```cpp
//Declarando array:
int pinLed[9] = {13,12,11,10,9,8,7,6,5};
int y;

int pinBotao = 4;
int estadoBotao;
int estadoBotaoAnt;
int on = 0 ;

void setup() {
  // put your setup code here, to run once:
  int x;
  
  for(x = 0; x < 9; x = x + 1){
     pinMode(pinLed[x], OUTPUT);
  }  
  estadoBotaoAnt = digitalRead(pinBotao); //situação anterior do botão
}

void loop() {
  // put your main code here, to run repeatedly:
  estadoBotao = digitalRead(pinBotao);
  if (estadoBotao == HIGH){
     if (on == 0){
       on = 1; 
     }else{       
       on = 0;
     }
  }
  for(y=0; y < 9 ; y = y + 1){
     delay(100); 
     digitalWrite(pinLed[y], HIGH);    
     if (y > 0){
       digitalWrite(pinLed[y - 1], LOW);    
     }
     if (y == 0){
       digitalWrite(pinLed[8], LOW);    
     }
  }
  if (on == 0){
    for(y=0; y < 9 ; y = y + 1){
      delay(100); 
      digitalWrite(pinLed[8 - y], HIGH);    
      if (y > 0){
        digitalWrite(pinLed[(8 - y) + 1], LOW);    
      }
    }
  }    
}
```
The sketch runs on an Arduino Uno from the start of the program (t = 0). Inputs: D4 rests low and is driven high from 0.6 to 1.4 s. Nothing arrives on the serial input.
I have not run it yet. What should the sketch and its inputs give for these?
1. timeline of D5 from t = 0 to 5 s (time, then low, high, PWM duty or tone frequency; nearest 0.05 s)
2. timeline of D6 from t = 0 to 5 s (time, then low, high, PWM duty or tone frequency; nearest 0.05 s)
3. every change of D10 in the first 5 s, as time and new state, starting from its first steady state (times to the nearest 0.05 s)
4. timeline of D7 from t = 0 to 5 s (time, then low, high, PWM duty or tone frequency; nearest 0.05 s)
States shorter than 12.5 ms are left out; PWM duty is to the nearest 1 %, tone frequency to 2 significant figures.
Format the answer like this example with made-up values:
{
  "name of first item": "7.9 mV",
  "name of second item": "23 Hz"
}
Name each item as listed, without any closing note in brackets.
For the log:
{
  "timeline of D5 from t = 0 to 5 s": "0 s low; 0.9 s high; 1.1 s low; 2.7 s high; 2.9 s low; 4.5 s high; 4.7 s low",
  "timeline of D6 from t = 0 to 5 s": "0 s low; 0.8 s high; 0.9 s low; 1.1 s high; 1.2 s low; 2.6 s high; 2.7 s low; 2.9 s high; 3 s low; 4.4 s high; 4.5 s low; 4.7 s high; 4.8 s low",
  "every change of D10 in the first 5 s, as time and new state, starting from its first steady state": "0 s low; 0.4 s high; 0.5 s low; 1.5 s high; 1.6 s low; 2.2 s high; 2.3 s low; 3.3 s high; 3.4 s low; 4 s high; 4.1 s low",
  "timeline of D7 from t = 0 to 5 s": "0 s low; 0.7 s high; 0.8 s low; 1.2 s high; 1.3 s low; 2.5 s high; 2.6 s low; 3 s high; 3.1 s low; 4.3 s high; 4.4 s low; 4.8 s high; 4.9 s low"
}
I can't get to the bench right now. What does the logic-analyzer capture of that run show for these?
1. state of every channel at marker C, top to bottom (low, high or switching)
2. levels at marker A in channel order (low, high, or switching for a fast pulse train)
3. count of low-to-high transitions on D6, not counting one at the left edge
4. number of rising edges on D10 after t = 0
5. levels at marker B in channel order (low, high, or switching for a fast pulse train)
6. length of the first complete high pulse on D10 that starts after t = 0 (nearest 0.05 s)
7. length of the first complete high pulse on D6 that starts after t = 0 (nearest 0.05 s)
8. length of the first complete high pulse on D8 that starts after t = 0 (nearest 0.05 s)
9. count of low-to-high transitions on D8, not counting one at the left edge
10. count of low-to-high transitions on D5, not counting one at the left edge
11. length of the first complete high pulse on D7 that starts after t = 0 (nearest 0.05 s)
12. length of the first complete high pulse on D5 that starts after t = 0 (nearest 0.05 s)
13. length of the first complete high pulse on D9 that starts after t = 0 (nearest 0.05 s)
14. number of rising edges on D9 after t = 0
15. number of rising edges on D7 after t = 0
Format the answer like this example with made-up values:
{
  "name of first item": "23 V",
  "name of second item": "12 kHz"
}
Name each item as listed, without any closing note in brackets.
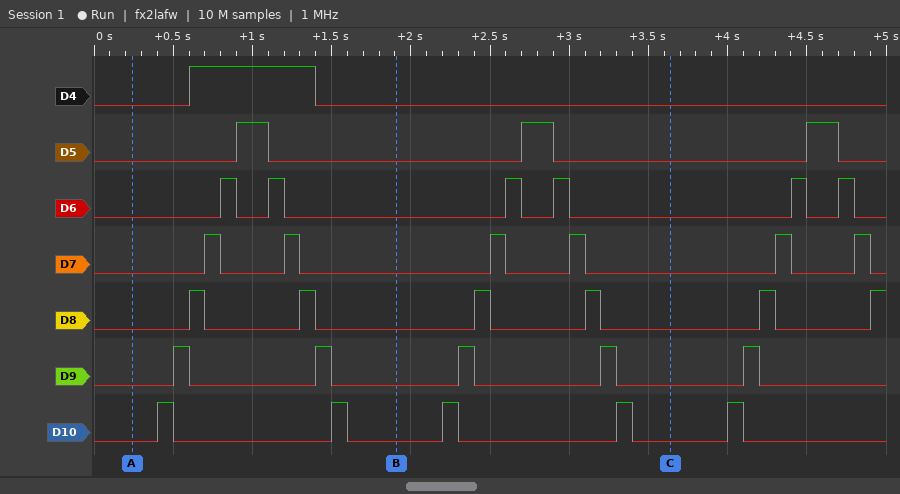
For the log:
{
  "state of every channel at marker C, top to bottom": "D4 low, D5 low, D6 low, D7 low, D8 low, D9 low, D10 low",
  "levels at marker A in channel order": "D4 low, D5 low, D6 low, D7 low, D8 low, D9 low, D10 low",
  "count of low-to-high transitions on D6, not counting one at the left edge": "6",
  "number of rising edges on D10 after t = 0": "5",
  "levels at marker B in channel order": "D4 low, D5 low, D6 low, D7 low, D8 low, D9 low, D10 low",
  "length of the first complete high pulse on D10 that starts after t = 0": "0.10 s",
  "length of the first complete high pulse on D6 that starts after t = 0": "0.10 s",
  "length of the first complete high pulse on D8 that starts after t = 0": "0.10 s",
  "count of low-to-high transitions on D8, not counting one at the left edge": "6",
  "count of low-to-high transitions on D5, not counting one at the left edge": "3",
  "length of the first complete high pulse on D7 that starts after t = 0": "0.10 s",
  "length of the first complete high pulse on D5 that starts after t = 0": "0.20 s",
  "length of the first complete high pulse on D9 that starts after t = 0": "0.10 s",
  "number of rising edges on D9 after t = 0": "5",
  "number of rising edges on D7 after t = 0": "6"
}
